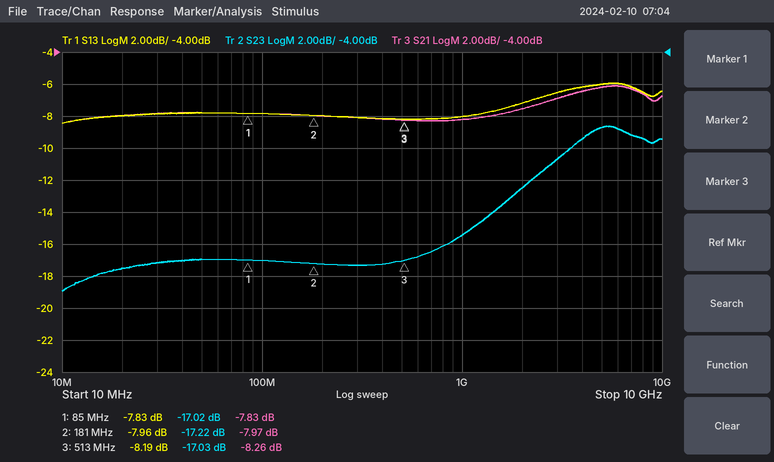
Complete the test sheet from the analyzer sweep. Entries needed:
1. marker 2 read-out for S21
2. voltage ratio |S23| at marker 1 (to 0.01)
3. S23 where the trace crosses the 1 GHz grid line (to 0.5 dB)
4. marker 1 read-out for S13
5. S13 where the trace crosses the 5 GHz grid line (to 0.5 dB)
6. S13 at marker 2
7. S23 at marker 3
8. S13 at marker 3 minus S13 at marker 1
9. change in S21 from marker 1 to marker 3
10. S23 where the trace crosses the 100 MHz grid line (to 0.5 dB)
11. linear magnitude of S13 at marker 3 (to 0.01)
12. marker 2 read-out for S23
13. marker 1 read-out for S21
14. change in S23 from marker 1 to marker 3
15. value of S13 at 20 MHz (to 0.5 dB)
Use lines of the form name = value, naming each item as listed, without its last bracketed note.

marker 2 read-out for S21 = -7.97 dB
voltage ratio |S23| at marker 1 = 0.14
S23 where the trace crosses the 1 GHz grid line = -15.5 dB
marker 1 read-out for S13 = -7.83 dB
S13 where the trace crosses the 5 GHz grid line = -6.0 dB
S13 at marker 2 = -7.96 dB
S23 at marker 3 = -17.03 dB
S13 at marker 3 minus S13 at marker 1 = -0.36 dB
change in S21 from marker 1 to marker 3 = -0.43 dB
S23 where the trace crosses the 100 MHz grid line = -17.0 dB
linear magnitude of S13 at marker 3 = 0.39
marker 2 read-out for S23 = -17.22 dB
marker 1 read-out for S21 = -7.83 dB
change in S23 from marker 1 to marker 3 = -0.01 dB
value of S13 at 20 MHz = -8.0 dB
